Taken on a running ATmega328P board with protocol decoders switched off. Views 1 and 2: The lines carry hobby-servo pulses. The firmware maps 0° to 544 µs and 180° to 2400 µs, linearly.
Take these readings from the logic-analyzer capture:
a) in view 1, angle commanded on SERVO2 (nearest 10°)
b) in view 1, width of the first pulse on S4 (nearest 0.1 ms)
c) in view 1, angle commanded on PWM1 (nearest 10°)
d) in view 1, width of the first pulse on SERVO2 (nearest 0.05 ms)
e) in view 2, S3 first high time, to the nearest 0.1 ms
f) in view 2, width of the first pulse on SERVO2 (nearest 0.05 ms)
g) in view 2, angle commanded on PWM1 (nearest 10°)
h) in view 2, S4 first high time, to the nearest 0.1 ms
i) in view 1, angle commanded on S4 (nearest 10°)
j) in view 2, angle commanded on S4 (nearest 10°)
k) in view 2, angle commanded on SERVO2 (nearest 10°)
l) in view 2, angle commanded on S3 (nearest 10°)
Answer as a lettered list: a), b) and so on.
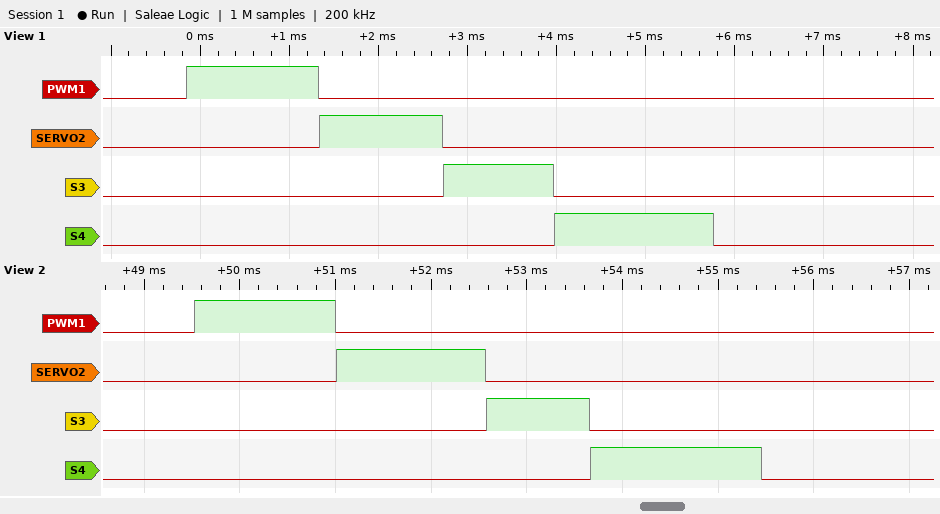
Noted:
a) 80°
b) 1.8 ms
c) 90°
d) 1.40 ms
e) 1.1 ms
f) 1.55 ms
g) 90°
h) 1.8 ms
i) 120°
j) 120°
k) 100°
l) 50°
